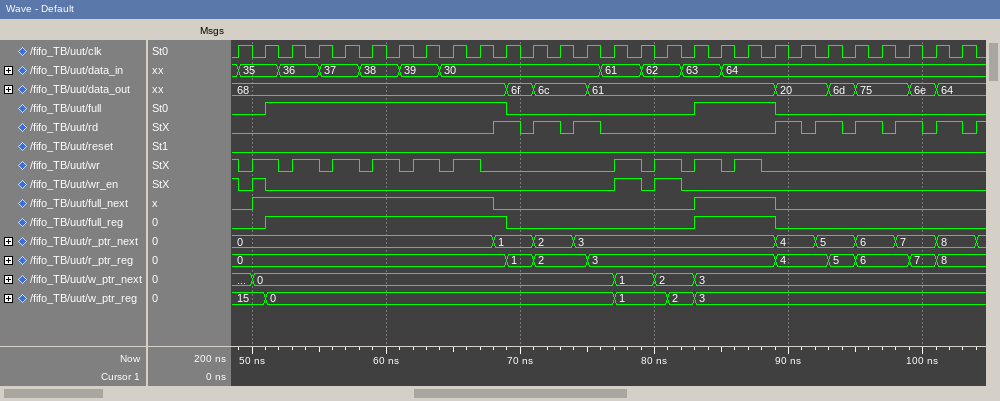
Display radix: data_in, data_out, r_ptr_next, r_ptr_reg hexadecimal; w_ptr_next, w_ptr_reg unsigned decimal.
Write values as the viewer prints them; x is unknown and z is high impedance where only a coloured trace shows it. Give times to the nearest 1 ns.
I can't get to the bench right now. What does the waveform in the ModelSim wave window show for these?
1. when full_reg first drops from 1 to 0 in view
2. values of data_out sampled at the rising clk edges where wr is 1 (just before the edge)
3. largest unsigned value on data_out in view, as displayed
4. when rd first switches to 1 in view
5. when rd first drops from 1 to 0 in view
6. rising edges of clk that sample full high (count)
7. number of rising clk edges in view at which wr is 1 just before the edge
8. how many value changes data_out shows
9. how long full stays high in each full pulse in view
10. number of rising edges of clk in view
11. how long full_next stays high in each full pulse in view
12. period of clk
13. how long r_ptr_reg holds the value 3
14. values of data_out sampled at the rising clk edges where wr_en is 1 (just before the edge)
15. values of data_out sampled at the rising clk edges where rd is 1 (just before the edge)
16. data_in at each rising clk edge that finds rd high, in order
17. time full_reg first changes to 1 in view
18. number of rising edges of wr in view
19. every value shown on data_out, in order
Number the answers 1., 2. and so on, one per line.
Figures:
1. 69 ns
2. 68, 68, 68, 68, 68, 68, 68, 61, 61, 61, 61
3. 75
4. 68 ns
5. 70 ns
6. 12
7. 11
8. 8
9. 18 ns, 6 ns
10. 28
11. 18 ns, 6 ns
12. 2 ns
13. 14 ns
14. 68, 68, 61, 61
15. 68, 6c, 6c, 20, 20, 75, 75, 64
16. 30, 30, 30, 64, 64, 64, 64, 64
17. 51 ns
18. 10
19. 68, 6f, 6c, 61, 20, 6d, 75, 6e, 64
